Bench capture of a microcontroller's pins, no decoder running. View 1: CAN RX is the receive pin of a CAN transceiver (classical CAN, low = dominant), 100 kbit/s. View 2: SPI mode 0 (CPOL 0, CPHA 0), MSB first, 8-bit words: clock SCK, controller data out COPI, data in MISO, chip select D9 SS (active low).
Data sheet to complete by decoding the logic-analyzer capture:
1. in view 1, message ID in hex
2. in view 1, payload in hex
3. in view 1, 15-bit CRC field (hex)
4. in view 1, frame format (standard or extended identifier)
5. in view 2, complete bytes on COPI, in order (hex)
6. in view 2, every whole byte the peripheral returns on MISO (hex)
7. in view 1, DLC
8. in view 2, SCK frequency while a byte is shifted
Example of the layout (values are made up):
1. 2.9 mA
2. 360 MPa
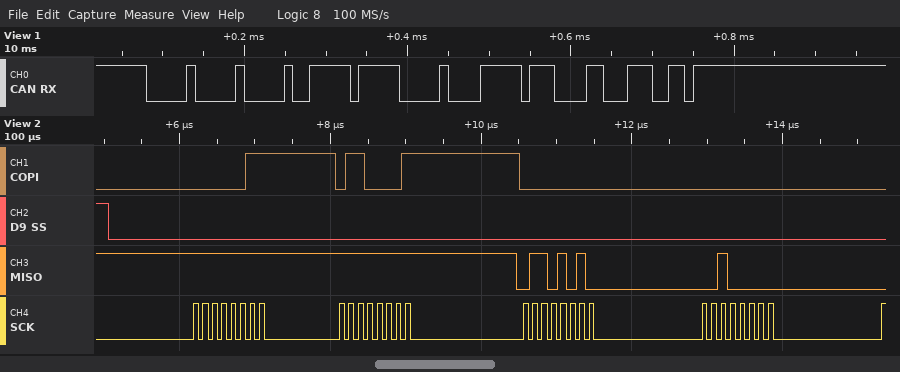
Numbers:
1. 0x000
2. FF 00 FF
3. 0x0639
4. standard
5. 0x03 0x61 0x00 0x00
6. 0xFF 0xFF 0x6A 0x20
7. 3
8. 8 MHz
